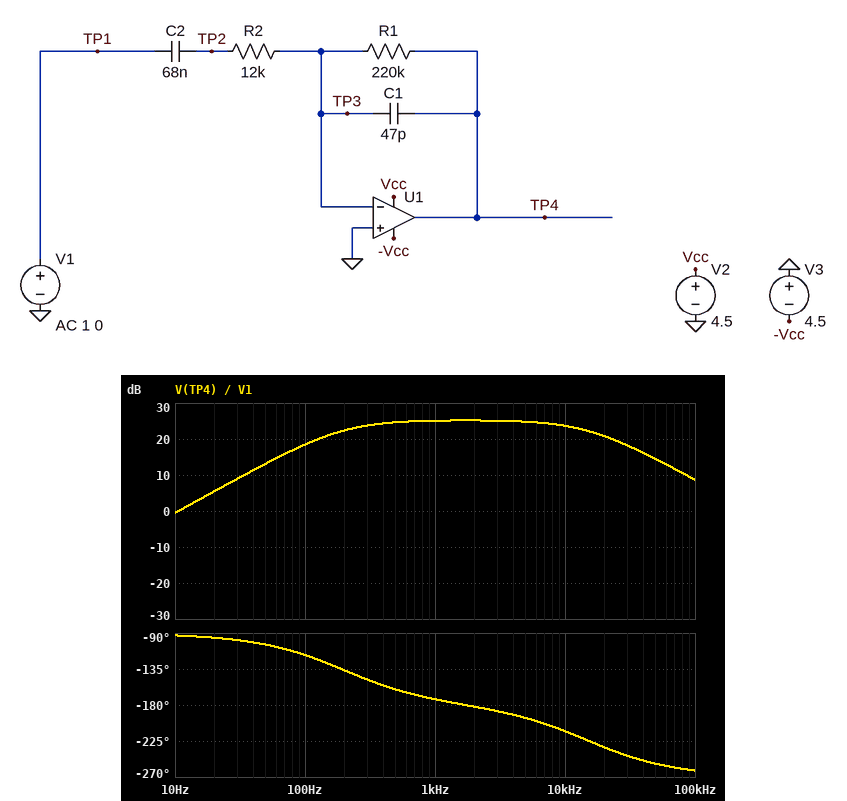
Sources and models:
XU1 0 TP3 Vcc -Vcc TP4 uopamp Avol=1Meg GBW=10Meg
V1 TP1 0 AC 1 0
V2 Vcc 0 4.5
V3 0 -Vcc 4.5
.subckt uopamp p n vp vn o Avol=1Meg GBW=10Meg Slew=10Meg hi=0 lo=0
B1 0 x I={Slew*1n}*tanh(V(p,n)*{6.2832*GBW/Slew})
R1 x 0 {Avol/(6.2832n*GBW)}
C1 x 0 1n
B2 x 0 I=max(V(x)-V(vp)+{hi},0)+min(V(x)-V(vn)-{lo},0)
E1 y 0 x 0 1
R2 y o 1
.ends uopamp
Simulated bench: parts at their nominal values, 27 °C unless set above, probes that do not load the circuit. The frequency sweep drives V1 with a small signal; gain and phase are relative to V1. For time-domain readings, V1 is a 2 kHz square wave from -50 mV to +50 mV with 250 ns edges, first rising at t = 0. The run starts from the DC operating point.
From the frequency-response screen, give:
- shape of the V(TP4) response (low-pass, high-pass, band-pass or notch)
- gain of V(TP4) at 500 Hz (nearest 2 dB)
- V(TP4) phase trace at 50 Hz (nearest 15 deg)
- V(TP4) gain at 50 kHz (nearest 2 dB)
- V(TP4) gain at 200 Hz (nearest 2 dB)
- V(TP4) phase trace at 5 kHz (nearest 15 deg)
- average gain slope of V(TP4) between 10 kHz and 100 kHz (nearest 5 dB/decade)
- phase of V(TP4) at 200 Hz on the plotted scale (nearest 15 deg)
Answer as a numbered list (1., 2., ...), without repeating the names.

1. band-pass
2. 24 dB
3. -105 deg
4. 14 dB
5. 22 dB
6. -195 deg
7. -15 dB/decade
8. -135 deg
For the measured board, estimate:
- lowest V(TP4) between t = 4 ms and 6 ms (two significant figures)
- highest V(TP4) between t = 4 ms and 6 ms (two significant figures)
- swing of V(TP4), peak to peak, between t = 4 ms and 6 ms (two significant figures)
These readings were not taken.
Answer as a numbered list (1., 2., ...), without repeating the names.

1. -1.0 V
2. 990 mV
3. 2.0 V
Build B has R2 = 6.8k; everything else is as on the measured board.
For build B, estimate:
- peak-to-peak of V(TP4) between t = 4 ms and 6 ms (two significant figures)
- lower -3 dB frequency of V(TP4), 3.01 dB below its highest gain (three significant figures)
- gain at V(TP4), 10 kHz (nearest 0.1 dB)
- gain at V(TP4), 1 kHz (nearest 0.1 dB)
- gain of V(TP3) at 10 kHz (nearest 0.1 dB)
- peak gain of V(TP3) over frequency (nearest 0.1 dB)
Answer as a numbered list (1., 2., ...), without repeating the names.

1. 3.7 V
2. 329 Hz
3. 28.5 dB
4. 29.7 dB
5. -31.5 dB
6. -26.5 dB
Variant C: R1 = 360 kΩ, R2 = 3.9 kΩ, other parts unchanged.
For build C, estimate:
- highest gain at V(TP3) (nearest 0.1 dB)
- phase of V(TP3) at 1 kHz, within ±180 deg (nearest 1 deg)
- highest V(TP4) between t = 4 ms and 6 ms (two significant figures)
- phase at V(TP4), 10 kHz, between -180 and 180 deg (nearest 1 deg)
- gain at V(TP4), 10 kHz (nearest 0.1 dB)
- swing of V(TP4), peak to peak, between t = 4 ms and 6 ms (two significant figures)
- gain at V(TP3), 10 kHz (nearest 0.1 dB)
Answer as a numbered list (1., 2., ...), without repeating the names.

1. -22.0 dB
2. 114 deg
3. 4.5 V
4. 134 deg
5. 35.6 dB
6. 9.0 V
7. -24.4 dB
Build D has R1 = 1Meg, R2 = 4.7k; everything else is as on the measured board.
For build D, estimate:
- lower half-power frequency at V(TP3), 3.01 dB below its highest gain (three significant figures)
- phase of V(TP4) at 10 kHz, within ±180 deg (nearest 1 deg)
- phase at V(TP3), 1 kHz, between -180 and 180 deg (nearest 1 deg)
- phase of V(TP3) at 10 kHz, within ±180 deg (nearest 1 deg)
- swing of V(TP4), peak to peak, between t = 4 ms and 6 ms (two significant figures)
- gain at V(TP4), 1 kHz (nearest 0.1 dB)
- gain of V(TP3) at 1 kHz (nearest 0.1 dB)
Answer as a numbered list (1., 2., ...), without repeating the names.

1. 3.20 kHz
2. 110 deg
3. 98 deg
4. 20 deg
5. 9.0 V
6. 45.3 dB
7. -34.7 dB
